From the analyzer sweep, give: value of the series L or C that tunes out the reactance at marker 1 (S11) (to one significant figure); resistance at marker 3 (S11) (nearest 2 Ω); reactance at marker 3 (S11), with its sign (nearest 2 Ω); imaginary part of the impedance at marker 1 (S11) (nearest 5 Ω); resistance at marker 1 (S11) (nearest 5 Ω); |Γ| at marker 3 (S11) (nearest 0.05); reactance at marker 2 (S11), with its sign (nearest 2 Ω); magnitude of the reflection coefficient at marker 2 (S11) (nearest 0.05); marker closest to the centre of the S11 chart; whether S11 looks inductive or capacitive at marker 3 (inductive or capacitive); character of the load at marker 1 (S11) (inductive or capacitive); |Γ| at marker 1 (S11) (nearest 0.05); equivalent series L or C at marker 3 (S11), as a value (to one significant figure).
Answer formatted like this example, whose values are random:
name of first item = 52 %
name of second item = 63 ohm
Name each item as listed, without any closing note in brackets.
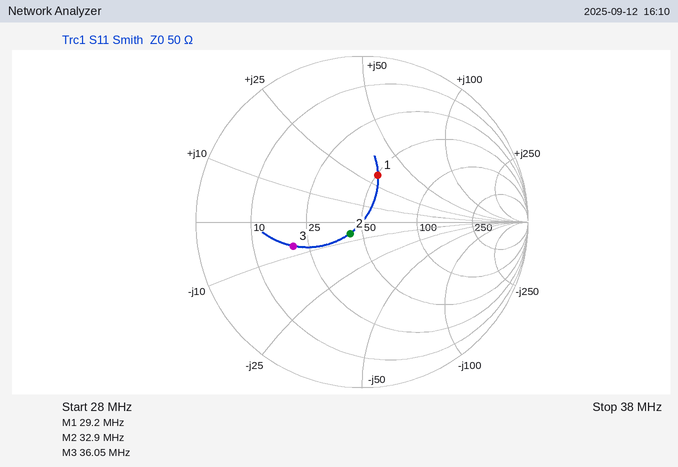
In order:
value of the series L or C that tunes out the reactance at marker 1 (S11) = 200 pF
resistance at marker 3 (S11) = 20 Ω
reactance at marker 3 (S11), with its sign = -8 Ω
imaginary part of the impedance at marker 1 (S11) = +30 Ω
resistance at marker 1 (S11) = 50 Ω
|Γ| at marker 3 (S11) = 0.45
reactance at marker 2 (S11), with its sign = -6 Ω
magnitude of the reflection coefficient at marker 2 (S11) = 0.10
marker closest to the centre of the S11 chart = marker 2
whether S11 looks inductive or capacitive at marker 3 = capacitive
character of the load at marker 1 (S11) = inductive
|Γ| at marker 1 (S11) = 0.30
equivalent series L or C at marker 3 (S11), as a value = 600 pF
